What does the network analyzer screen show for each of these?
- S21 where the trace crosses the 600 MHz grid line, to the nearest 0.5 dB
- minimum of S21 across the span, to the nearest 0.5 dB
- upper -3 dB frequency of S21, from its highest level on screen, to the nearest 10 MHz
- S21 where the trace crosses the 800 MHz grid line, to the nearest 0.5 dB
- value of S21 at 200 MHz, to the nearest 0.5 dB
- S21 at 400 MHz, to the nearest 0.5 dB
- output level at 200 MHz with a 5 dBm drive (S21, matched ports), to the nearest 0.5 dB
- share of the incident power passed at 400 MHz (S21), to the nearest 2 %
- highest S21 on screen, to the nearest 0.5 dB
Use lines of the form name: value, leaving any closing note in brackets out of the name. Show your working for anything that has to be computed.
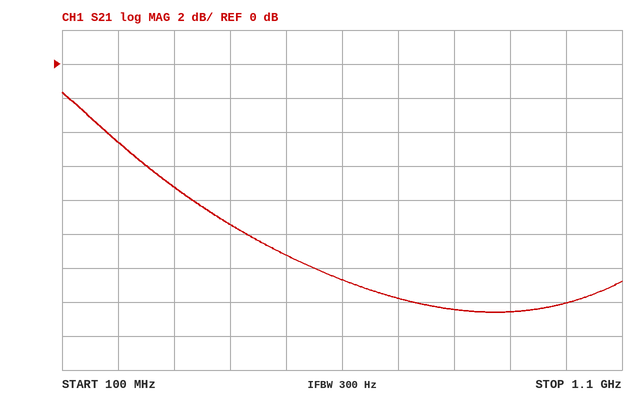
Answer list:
S21 where the trace crosses the 600 MHz grid line, to the nearest 0.5 dB: -12.5 dB
minimum of S21 across the span, to the nearest 0.5 dB: -14.5 dB
upper -3 dB frequency of S21, from its highest level on screen, to the nearest 10 MHz: 200 MHz
S21 where the trace crosses the 800 MHz grid line, to the nearest 0.5 dB: -14.5 dB
value of S21 at 200 MHz, to the nearest 0.5 dB: -4.5 dB
S21 at 400 MHz, to the nearest 0.5 dB: -9.5 dB
output level at 200 MHz with a 5 dBm drive (S21, matched ports), to the nearest 0.5 dB: 5 dBm + (-4.5 dB) = 0.5 dBm
share of the incident power passed at 400 MHz (S21), to the nearest 2 %: 10^(-9.5/10) ≈ 11.2 %, so 12 % to the nearest 2 %
highest S21 on screen, to the nearest 0.5 dB: -1.5 dB
